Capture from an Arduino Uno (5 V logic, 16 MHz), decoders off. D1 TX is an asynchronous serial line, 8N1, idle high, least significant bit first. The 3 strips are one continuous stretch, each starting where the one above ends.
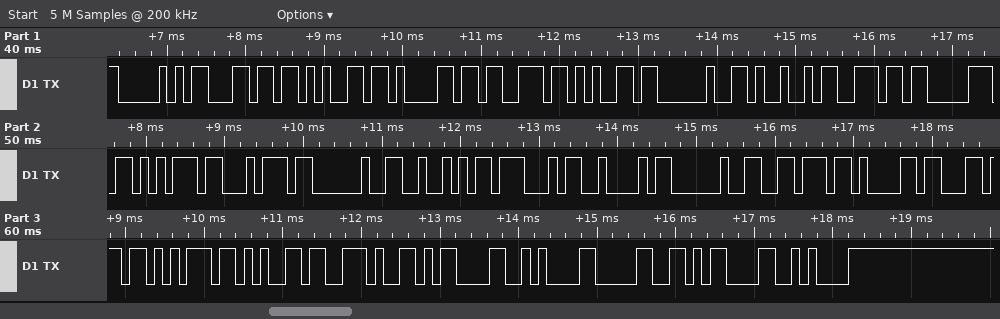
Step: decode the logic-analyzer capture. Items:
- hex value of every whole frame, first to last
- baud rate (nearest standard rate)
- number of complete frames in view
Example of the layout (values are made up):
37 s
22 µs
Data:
50 6C 65 61 73 65 20 49 6E 70 75 74 20 52 47 42 20 76 61 6C 75 65 2E 0D 0A 30 0D 0A
9600 baud
28
